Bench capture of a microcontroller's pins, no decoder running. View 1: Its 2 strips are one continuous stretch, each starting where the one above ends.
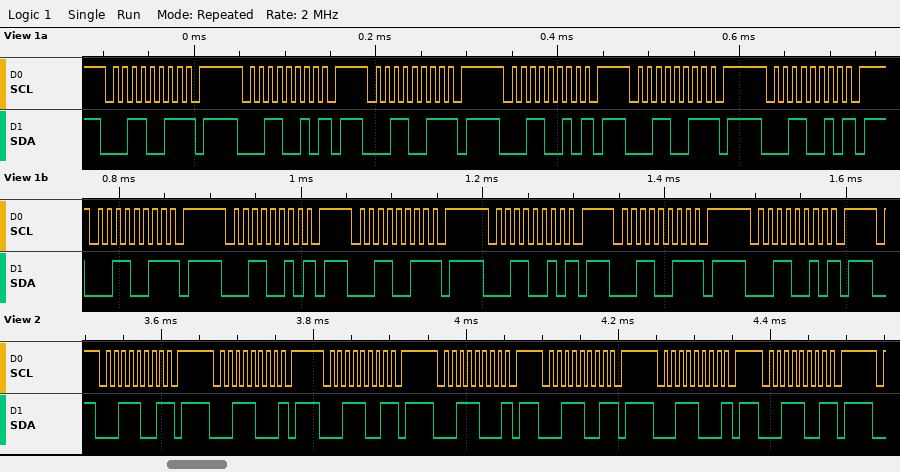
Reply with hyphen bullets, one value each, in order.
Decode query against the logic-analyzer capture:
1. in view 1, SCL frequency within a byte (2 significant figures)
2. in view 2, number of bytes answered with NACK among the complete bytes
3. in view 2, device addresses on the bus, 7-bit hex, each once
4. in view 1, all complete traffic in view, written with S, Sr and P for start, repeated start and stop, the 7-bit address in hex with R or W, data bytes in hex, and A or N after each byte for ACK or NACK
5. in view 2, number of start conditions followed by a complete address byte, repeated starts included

- 100 kHz
- 7
- 0x1C
- S 19R N P S 19W N P S 19R N P S 19W N P S 19R N P S 19W N P S 19R N P S 19W N P S 19R N P S 19W N P S 19R N P S 19W N P
- 7
